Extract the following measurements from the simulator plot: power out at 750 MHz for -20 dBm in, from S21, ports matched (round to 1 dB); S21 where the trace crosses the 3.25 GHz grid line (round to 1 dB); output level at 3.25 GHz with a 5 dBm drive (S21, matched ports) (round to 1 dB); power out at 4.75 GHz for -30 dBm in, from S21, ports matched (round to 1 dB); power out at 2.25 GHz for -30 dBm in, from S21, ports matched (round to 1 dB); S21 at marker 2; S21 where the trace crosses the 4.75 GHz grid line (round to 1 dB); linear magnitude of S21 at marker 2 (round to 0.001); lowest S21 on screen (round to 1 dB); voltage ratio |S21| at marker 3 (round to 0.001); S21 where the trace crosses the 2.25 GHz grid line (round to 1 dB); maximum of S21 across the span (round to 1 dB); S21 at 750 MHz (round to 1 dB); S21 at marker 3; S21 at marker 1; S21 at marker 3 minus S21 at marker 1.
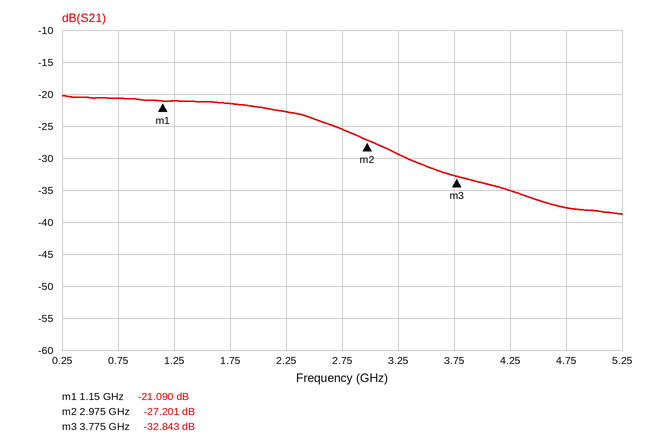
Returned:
-41 dBm
-29 dB
-24 dBm
-68 dBm
-53 dBm
-27.201 dB
-38 dB
0.044
-39 dB
0.023
-23 dB
-20 dB
-21 dB
-32.843 dB
-21.090 dB
-11.753 dB
